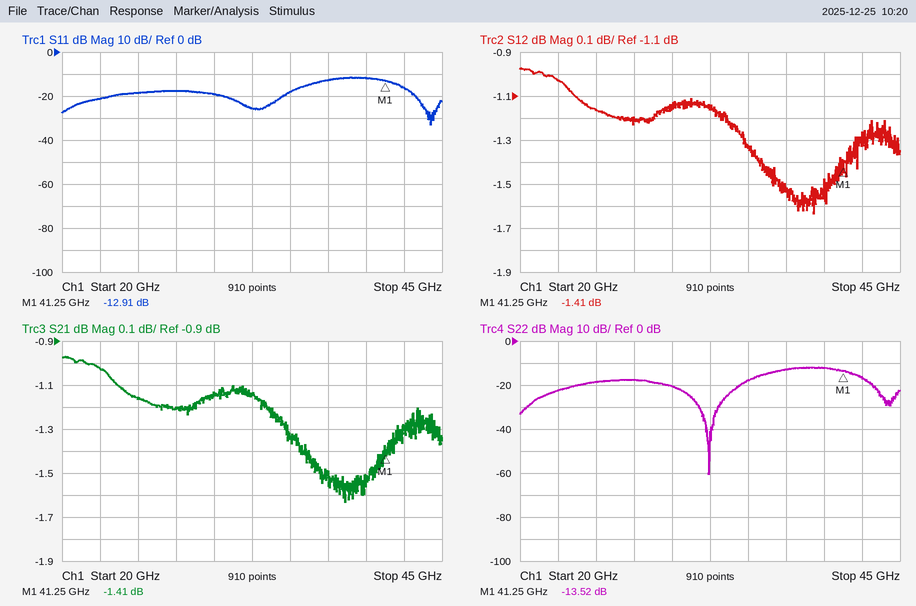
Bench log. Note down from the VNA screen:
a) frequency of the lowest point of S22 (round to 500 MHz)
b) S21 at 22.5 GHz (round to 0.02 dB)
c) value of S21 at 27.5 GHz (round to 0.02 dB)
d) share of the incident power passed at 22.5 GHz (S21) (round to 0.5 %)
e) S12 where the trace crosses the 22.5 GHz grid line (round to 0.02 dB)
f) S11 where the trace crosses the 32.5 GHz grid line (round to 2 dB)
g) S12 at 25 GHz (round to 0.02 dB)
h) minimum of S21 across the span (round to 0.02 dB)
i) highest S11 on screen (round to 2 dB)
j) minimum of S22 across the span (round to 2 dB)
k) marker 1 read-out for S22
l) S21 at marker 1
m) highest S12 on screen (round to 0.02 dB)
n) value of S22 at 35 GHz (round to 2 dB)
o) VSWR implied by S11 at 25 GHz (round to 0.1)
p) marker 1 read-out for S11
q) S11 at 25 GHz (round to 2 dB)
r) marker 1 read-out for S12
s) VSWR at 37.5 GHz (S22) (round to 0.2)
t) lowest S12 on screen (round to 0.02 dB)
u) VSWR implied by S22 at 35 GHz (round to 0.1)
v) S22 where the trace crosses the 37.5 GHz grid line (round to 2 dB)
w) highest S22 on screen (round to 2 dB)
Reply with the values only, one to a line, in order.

32.5 GHz
-1.02 dB
-1.20 dB
79.0 %
-1.02 dB
-26 dB
-1.16 dB
-1.64 dB
-12 dB
-60 dB
-13.52 dB
-1.41 dB
-0.98 dB
-18 dB
1.3
-12.91 dB
-18 dB
-1.41 dB
1.6
-1.64 dB
1.3
-12 dB
-12 dB
